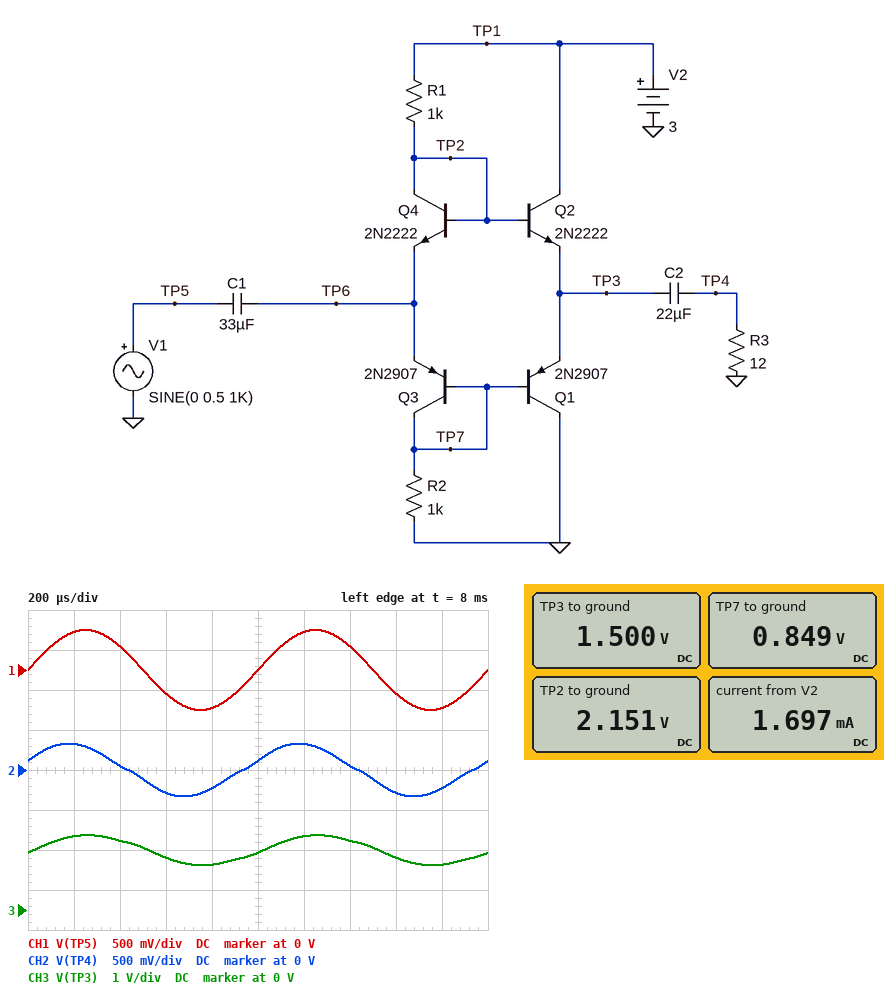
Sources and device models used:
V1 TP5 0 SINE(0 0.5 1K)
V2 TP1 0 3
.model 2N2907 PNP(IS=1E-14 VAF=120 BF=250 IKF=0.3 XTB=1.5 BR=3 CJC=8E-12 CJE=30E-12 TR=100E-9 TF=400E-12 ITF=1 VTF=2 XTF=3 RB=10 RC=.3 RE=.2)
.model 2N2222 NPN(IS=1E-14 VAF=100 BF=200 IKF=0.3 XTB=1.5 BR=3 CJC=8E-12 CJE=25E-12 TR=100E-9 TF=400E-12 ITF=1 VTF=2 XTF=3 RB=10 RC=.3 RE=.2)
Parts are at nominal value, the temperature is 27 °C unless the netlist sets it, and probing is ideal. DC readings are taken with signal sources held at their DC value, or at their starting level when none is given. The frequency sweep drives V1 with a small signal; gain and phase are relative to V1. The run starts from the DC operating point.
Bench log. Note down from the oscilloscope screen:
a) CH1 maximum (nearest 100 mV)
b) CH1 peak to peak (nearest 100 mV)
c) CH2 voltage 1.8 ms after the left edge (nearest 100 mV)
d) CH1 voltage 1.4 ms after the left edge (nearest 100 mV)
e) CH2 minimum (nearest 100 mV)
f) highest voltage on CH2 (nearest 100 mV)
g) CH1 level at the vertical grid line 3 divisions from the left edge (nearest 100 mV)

500 mV
1.0 V
-200 mV
300 mV
-300 mV
300 mV
-300 mV
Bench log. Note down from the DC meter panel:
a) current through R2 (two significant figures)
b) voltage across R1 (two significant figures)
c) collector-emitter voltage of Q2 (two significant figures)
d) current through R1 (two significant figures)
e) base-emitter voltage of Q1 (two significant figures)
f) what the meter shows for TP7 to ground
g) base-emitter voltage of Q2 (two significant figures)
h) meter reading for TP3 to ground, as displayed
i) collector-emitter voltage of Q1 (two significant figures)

850 µA
850 mV
1.5 V
850 µA
-650 mV
0.849 V
650 mV
1.500 V
-1.5 V
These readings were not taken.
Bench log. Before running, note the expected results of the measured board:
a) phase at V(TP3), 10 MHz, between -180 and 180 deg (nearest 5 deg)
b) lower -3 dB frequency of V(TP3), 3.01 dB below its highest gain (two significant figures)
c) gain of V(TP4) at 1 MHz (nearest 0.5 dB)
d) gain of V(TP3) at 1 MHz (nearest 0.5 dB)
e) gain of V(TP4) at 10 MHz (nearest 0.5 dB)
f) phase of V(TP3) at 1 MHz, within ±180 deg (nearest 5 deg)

0 deg
8.8 Hz
-7.5 dB
-7.5 dB
-7.5 dB
0 deg
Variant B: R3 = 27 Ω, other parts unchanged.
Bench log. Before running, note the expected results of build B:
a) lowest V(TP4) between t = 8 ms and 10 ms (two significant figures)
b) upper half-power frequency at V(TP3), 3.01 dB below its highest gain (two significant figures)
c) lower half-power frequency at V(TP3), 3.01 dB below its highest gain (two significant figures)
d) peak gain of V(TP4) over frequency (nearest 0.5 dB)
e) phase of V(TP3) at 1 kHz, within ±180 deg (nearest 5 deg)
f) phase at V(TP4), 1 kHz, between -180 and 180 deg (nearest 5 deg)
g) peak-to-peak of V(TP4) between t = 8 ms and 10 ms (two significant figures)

-390 mV
540 Hz
8.6 Hz
-4.0 dB
-5 deg
10 deg
770 mV
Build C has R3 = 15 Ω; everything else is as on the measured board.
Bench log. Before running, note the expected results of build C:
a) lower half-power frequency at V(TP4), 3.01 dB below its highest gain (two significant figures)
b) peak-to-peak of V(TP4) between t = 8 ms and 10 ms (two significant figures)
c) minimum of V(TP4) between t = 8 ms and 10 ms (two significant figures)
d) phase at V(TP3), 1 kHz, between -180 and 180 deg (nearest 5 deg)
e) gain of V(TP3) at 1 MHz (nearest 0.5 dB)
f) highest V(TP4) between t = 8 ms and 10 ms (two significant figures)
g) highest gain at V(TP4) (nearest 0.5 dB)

270 Hz
700 mV
-350 mV
-10 deg
-6.5 dB
350 mV
-6.0 dB
